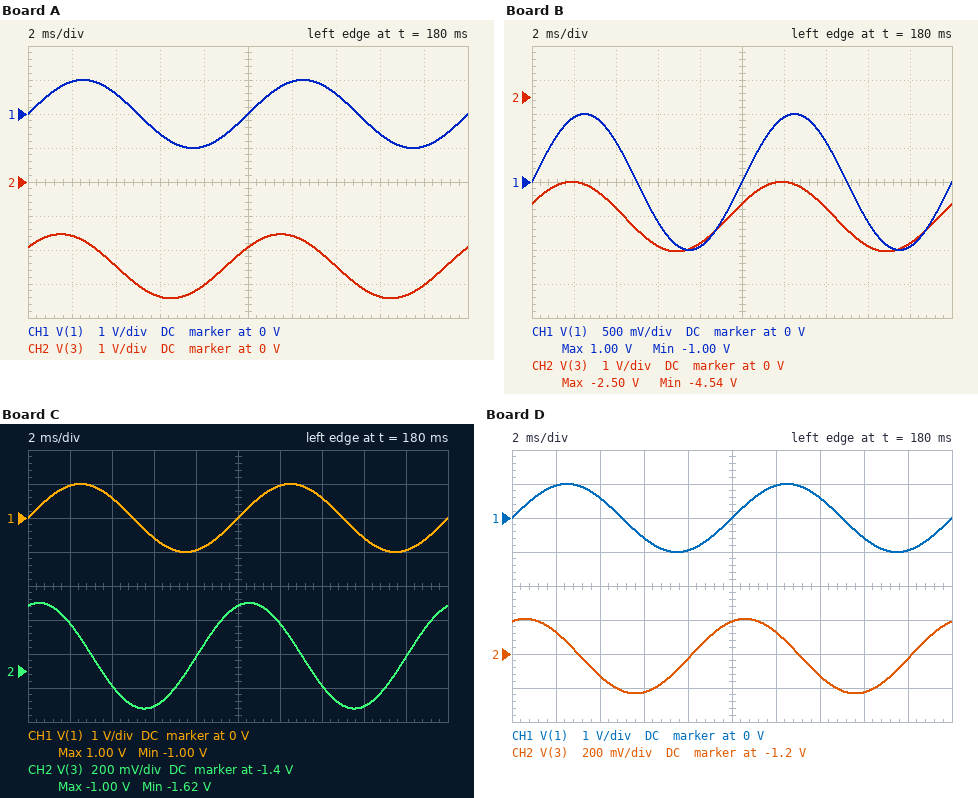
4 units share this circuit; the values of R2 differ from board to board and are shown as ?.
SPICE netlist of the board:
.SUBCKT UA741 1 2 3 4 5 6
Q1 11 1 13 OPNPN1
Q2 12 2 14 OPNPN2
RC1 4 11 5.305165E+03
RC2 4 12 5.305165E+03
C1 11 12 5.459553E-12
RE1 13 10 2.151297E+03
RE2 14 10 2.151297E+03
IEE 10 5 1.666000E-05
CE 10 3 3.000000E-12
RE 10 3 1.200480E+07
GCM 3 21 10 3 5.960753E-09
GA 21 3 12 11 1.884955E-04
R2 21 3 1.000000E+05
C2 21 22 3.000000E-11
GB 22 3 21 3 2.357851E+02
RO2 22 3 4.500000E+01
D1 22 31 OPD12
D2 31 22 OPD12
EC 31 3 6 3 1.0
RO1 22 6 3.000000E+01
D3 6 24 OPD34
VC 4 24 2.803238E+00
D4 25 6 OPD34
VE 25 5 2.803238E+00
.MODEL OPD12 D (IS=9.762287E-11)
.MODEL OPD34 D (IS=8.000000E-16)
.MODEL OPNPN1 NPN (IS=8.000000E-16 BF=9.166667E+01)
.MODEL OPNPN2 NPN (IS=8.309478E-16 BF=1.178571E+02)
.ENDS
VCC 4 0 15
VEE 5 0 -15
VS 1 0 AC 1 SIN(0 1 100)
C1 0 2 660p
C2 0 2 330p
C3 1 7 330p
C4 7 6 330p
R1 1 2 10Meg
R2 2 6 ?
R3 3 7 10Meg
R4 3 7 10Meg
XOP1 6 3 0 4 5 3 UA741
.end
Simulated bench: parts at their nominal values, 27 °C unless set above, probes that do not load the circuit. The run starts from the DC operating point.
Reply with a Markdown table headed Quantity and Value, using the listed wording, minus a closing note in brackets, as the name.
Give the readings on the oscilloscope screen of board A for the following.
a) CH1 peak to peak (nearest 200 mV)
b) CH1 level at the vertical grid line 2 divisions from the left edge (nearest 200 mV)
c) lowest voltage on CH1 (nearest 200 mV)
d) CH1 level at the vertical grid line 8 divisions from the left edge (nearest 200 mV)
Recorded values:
| Quantity | Value |
|---|---|
| CH1 peak to peak | 2.0 V |
| CH1 level at the vertical grid line 2 divisions from the left edge | 600 mV |
| lowest voltage on CH1 | -1.0 V |
| CH1 level at the vertical grid line 8 divisions from the left edge | -600 mV |
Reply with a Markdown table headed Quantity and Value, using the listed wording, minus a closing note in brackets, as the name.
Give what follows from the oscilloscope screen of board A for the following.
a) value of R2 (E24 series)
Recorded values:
| Quantity | Value |
|---|---|
| value of R2 | 18 MΩ |
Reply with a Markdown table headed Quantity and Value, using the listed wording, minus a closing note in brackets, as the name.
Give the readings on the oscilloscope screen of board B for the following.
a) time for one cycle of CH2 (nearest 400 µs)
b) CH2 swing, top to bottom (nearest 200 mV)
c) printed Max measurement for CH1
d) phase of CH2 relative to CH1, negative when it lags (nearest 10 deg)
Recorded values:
| Quantity | Value |
|---|---|
| time for one cycle of CH2 | 10.0 ms |
| CH2 swing, top to bottom | 2.0 V |
| printed Max measurement for CH1 | 1.00 V |
| phase of CH2 relative to CH1, negative when it lags | 20 deg |
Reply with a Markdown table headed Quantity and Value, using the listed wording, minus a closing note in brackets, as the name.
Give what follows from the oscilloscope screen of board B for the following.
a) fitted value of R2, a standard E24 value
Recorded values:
| Quantity | Value |
|---|---|
| fitted value of R2, a standard E24 value | 30 MΩ |
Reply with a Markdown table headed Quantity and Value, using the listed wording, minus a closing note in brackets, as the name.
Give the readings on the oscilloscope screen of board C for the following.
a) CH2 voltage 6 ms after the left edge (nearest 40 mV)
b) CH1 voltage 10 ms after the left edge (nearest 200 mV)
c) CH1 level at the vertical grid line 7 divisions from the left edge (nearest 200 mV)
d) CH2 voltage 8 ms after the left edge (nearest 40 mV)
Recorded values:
| Quantity | Value |
|---|---|
| CH2 voltage 6 ms after the left edge | -1.60 V |
| CH1 voltage 10 ms after the left edge | 0 V |
| CH1 level at the vertical grid line 7 divisions from the left edge | 600 mV |
| CH2 voltage 8 ms after the left edge | -1.32 V |
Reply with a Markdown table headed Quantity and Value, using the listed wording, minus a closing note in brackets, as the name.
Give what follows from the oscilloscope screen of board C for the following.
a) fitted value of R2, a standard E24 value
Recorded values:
| Quantity | Value |
|---|---|
| fitted value of R2, a standard E24 value | 4.7 MΩ |
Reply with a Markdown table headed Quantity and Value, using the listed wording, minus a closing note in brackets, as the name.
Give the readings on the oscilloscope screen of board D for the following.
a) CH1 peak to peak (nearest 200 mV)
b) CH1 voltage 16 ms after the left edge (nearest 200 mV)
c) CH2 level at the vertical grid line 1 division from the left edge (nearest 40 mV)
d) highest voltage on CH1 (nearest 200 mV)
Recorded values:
| Quantity | Value |
|---|---|
| CH1 peak to peak | 2.0 V |
| CH1 voltage 16 ms after the left edge | -600 mV |
| CH2 level at the vertical grid line 1 division from the left edge | -1.08 V |
| highest voltage on CH1 | 1.0 V |
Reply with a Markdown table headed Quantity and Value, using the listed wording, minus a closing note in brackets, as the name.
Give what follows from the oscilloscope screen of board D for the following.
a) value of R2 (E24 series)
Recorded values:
| Quantity | Value |
|---|---|
| value of R2 | 3.6 MΩ |
